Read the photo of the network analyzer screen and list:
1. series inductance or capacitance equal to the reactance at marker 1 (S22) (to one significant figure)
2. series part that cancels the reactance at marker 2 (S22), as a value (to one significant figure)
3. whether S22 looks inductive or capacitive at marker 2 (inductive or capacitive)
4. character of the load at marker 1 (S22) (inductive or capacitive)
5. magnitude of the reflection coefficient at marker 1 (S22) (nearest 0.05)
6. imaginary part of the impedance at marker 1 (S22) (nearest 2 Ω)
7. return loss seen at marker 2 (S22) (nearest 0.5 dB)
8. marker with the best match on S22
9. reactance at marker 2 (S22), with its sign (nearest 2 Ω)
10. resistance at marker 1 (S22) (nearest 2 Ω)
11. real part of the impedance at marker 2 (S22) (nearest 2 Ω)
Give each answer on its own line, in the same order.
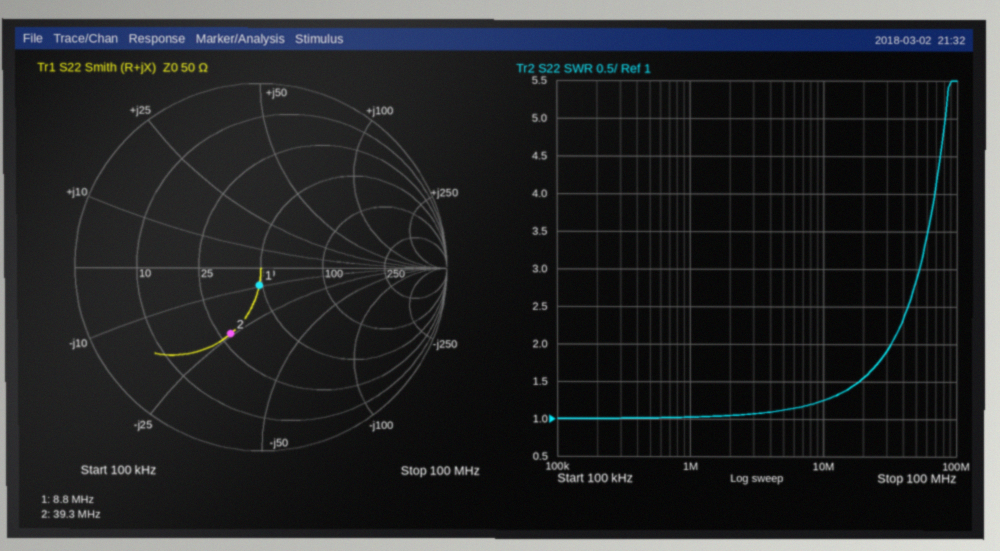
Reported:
2 nF
100 nH
capacitive
capacitive
0.10
-10 Ω
8.0 dB
marker 1
-24 Ω
48 Ω
28 Ω
